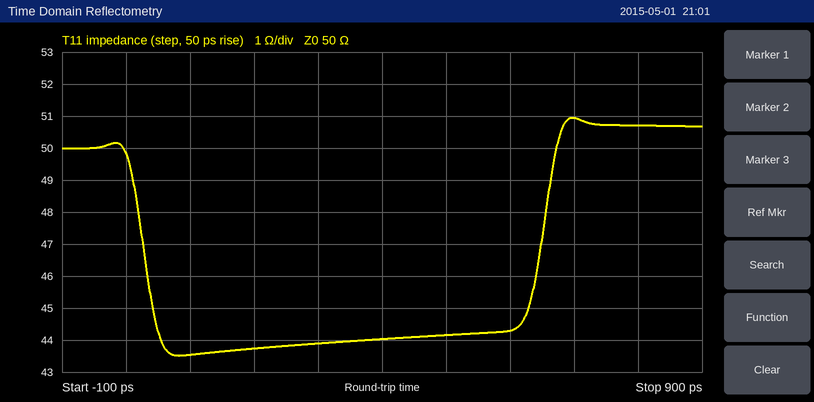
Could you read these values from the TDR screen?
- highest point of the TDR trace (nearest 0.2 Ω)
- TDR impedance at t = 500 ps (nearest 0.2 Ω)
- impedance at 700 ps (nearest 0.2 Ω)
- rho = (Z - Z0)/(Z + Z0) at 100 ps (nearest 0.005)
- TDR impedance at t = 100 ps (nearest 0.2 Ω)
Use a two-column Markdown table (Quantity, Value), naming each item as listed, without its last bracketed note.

| Quantity | Value |
|---|---|
| highest point of the TDR trace | 51.0 Ω |
| TDR impedance at t = 500 ps | 44.2 Ω |
| impedance at 700 ps | 51.0 Ω |
| rho = (Z - Z0)/(Z + Z0) at 100 ps | -0.070 |
| TDR impedance at t = 100 ps | 43.6 Ω |
